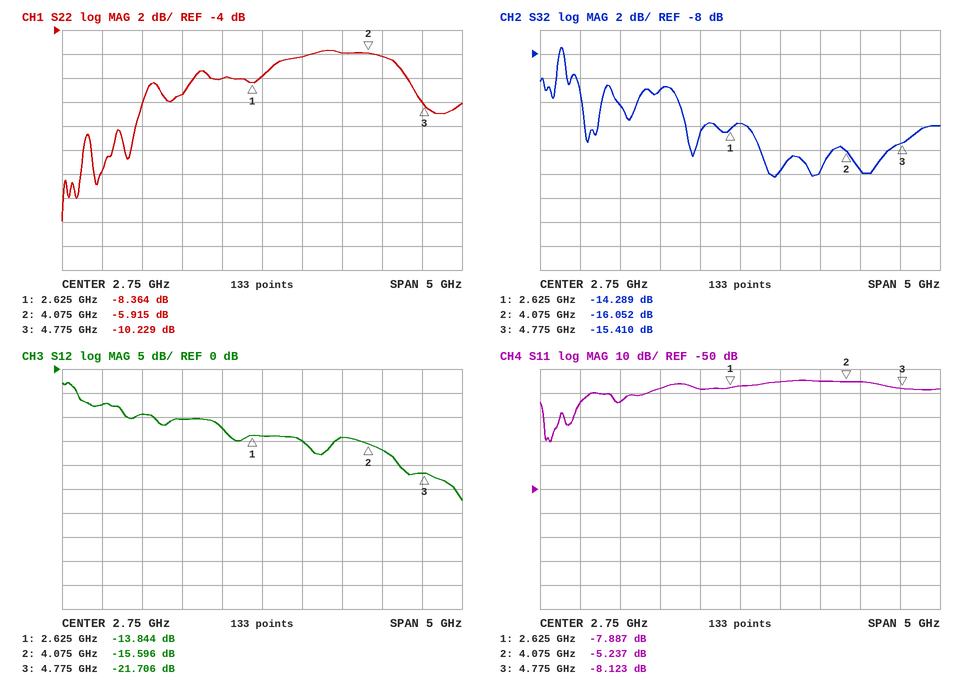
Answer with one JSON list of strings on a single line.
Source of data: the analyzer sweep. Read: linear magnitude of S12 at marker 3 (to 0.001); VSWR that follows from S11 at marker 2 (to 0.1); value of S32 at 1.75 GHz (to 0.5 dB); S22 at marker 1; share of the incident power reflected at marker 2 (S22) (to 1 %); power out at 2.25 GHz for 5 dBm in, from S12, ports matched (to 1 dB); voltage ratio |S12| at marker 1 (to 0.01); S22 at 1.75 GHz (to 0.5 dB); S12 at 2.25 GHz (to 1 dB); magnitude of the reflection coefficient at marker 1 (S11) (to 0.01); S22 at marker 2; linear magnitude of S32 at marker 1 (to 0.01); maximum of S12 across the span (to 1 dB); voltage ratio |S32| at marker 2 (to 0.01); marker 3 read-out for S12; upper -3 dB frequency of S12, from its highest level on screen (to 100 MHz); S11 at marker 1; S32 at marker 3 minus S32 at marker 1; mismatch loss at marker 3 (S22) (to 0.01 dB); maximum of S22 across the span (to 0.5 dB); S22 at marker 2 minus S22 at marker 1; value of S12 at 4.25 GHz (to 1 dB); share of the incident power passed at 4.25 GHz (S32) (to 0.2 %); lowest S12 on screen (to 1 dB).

["0.082", "3.4", "-11.0 dB", "-8.364 dB", "26 %", "-7 dBm", "0.20", "-9.5 dB", "-12 dB", "0.40", "-5.915 dB", "0.19", "-3 dB", "0.16", "-21.706 dB", "500 MHz", "-7.887 dB", "-1.121 dB", "0.43 dB", "-5.5 dB", "2.449 dB", "-17 dB", "1.8 %", "-27 dB"]
